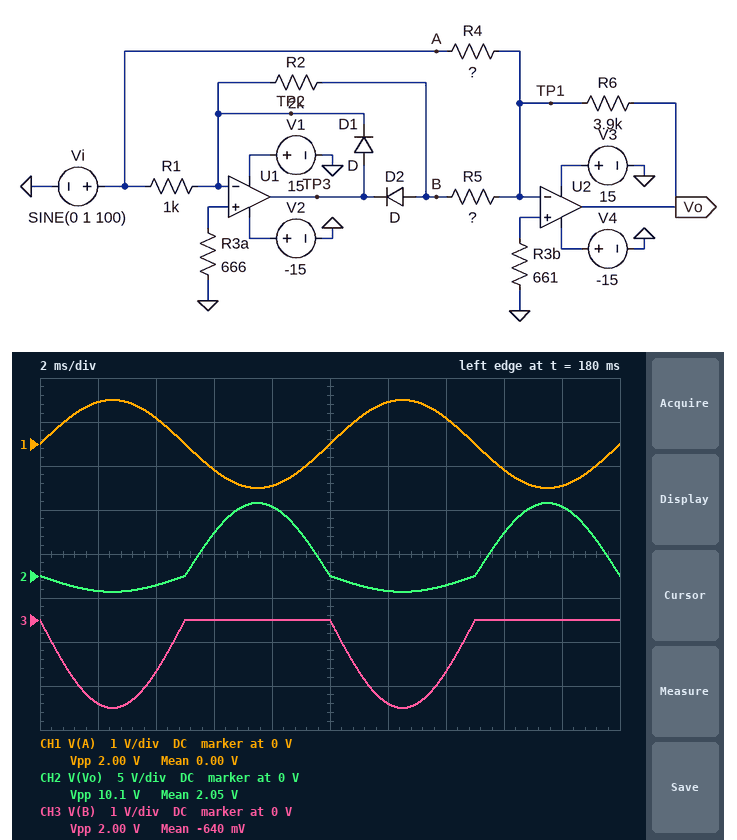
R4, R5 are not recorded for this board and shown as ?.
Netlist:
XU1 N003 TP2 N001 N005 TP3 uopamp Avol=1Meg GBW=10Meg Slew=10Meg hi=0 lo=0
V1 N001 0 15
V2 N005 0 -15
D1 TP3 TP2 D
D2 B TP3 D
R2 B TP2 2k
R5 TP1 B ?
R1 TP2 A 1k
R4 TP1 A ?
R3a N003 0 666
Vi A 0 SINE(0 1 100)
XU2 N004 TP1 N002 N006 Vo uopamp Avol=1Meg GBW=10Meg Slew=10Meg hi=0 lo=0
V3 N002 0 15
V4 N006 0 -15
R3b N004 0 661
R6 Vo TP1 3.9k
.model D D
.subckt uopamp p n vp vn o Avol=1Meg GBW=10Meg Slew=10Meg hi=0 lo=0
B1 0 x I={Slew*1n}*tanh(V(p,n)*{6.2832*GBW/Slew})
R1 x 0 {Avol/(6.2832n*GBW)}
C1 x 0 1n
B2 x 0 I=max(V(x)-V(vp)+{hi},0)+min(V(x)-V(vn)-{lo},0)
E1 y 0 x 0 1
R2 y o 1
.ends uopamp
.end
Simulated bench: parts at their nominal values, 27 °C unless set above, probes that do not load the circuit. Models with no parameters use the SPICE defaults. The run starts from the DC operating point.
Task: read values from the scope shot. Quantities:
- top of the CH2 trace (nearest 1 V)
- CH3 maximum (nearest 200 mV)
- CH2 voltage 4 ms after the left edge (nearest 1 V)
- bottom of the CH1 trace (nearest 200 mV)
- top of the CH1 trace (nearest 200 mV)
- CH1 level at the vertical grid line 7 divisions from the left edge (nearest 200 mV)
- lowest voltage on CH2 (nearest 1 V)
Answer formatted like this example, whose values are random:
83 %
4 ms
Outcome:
8 V
0 V
-1 V
-1.0 V
1.0 V
600 mV
-2 V
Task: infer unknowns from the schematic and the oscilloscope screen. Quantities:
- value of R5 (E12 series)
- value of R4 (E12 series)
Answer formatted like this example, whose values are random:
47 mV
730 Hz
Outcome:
1.2 kΩ
470 Ω
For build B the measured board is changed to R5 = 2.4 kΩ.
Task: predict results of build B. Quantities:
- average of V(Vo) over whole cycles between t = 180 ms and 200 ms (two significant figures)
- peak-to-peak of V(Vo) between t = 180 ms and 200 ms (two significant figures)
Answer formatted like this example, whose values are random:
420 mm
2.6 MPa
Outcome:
1.0 V
13 V
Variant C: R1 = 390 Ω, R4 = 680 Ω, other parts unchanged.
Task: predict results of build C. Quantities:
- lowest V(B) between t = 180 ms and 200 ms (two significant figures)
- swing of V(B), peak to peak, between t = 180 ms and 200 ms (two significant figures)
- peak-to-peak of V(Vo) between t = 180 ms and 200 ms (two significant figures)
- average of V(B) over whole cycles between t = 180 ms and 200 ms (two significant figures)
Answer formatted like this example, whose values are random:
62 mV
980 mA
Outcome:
-5.1 V
5.1 V
11 V
-1.6 V
